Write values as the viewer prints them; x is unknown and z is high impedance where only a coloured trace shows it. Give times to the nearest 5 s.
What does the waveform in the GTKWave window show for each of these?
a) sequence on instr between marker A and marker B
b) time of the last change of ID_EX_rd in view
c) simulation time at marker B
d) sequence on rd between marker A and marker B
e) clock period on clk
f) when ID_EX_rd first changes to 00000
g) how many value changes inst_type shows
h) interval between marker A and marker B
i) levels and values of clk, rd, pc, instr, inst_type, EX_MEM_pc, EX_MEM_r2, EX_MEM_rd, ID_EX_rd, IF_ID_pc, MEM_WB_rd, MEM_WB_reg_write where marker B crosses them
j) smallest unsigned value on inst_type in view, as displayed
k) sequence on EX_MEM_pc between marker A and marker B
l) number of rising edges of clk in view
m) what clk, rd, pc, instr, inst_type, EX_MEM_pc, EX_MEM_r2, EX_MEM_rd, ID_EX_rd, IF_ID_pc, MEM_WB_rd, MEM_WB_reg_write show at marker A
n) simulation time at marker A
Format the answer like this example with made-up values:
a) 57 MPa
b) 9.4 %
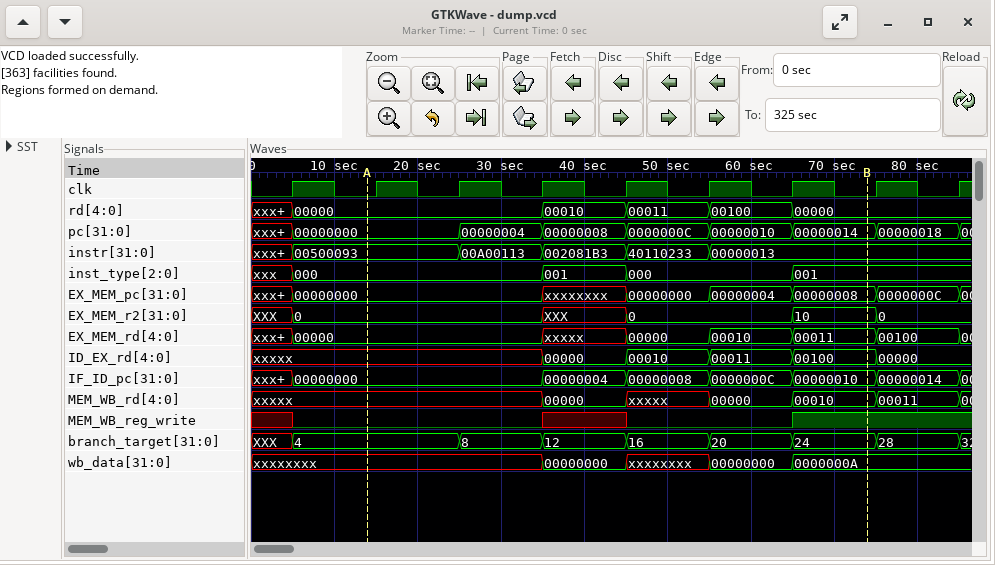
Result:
a) 00500093, 00A00113, 002081B3, 40110233, 00000013
b) 75 s
c) 75 s
d) 00000, 00010, 00011, 00100, 00000
e) 10 s
f) 35 s
g) 4
h) 60 s
i) clk=0, rd=00000, pc=00000014, instr=00000013, inst_type=001, EX_MEM_pc=00000008, EX_MEM_r2=10, EX_MEM_rd=00011, ID_EX_rd=00100, IF_ID_pc=00000010, MEM_WB_rd=00010, MEM_WB_reg_write=1
j) 000
k) 00000000, xxxxxxxx, 00000000, 00000004, 00000008
l) 9
m) clk=0, rd=00000, pc=00000000, instr=00500093, inst_type=000, EX_MEM_pc=00000000, EX_MEM_r2=0, EX_MEM_rd=00000, ID_EX_rd=xxxxx, IF_ID_pc=00000000, MEM_WB_rd=xxxxx, MEM_WB_reg_write=0
n) 15 s
